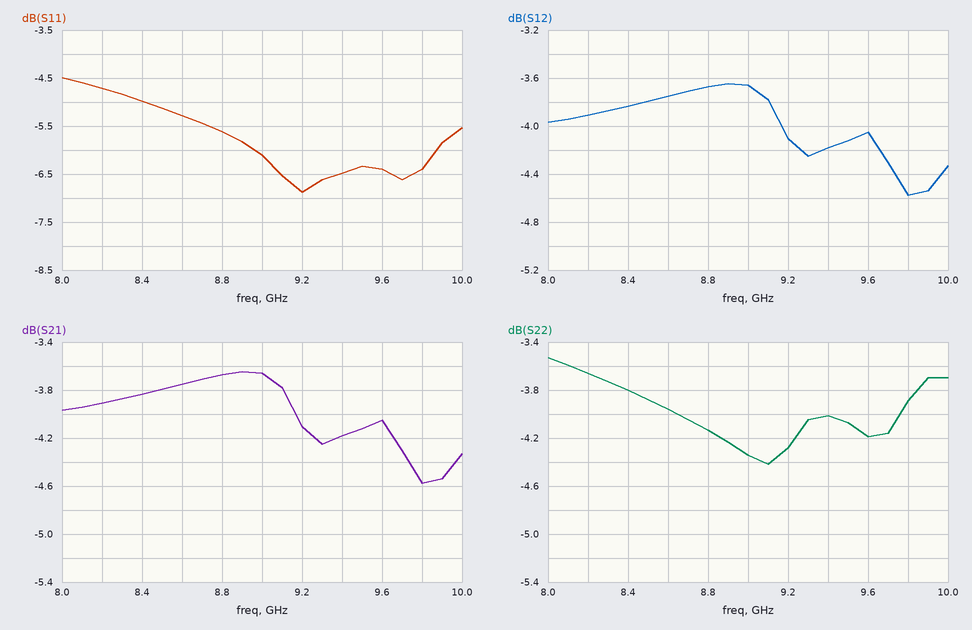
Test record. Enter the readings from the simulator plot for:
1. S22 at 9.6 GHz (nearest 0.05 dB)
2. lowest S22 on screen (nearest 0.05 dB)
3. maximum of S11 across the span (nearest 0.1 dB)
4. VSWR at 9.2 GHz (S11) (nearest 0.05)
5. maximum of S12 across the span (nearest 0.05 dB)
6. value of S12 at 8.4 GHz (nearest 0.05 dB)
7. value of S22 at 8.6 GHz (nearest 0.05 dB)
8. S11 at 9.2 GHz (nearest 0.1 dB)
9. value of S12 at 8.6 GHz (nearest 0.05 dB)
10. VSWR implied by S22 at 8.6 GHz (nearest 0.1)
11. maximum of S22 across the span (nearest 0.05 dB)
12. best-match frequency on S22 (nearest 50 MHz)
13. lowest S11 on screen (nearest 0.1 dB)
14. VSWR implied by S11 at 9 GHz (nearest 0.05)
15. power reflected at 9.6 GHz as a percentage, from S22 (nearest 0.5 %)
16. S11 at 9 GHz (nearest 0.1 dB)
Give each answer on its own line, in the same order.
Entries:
-4.20 dB
-4.40 dB
-4.5 dB
2.65
-3.65 dB
-3.85 dB
-3.95 dB
-6.9 dB
-3.75 dB
4.5
-3.55 dB
9.10 GHz
-6.9 dB
2.95
38.0 %
-6.1 dB
